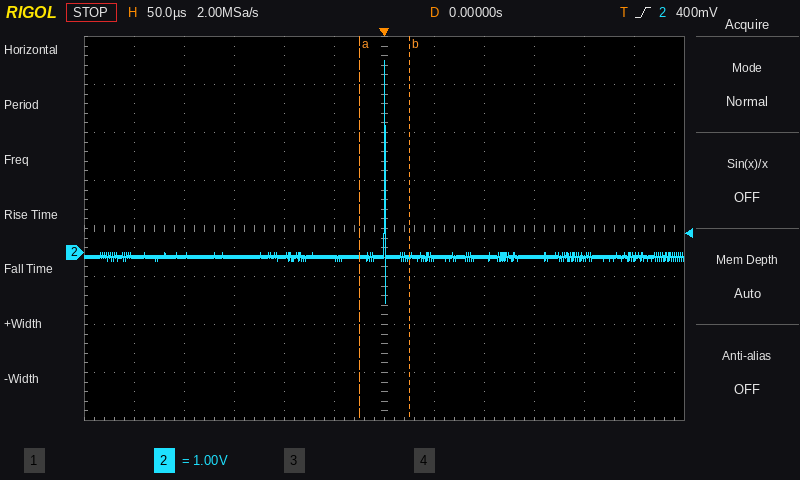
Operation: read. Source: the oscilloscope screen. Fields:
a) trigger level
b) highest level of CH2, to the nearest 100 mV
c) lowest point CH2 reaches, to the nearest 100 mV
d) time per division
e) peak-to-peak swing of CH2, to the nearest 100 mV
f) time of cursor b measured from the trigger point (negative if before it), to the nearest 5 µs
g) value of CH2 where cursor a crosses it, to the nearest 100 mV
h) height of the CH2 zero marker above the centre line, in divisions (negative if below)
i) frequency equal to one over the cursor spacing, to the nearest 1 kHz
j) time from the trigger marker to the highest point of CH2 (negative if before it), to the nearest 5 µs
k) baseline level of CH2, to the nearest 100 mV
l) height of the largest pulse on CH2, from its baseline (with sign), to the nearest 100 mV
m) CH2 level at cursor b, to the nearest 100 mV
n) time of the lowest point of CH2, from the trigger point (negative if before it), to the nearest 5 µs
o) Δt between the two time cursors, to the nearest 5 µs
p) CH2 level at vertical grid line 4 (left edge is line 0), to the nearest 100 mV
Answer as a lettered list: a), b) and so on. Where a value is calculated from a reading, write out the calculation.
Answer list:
a) 400 mV
b) 4.0 V
c) -1.1 V
d) 50 µs
e) 4.0 V − (-1.1 V) = 5.1 V
f) +25 µs
g) -100 mV
h) -0.5 div
i) 1 / 50 µs ≈ 20 kHz
j) 0 µs
k) -100 mV
l) 4.0 V − (-100 mV) = +4.1 V
m) -100 mV
n) 0 µs
o) 50 µs
p) -100 mV
